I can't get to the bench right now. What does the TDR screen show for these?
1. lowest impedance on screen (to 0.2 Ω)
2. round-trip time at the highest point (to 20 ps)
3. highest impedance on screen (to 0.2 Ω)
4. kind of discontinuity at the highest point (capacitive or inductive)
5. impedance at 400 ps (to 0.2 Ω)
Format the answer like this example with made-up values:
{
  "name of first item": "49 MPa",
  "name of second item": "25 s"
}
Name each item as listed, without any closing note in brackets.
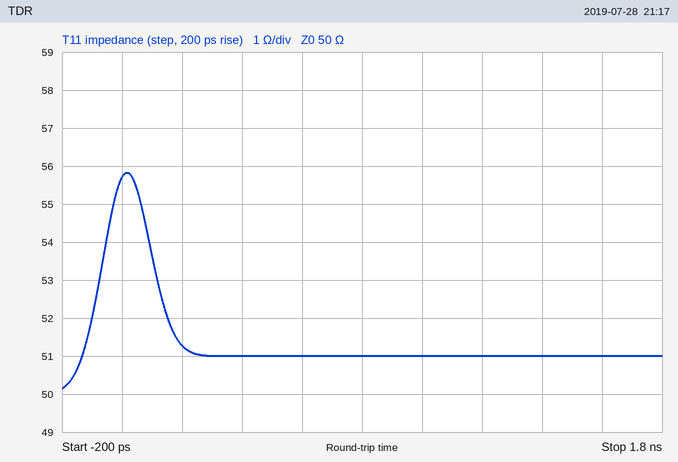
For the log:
{
  "lowest impedance on screen": "50.2 Ω",
  "round-trip time at the highest point": "20 ps",
  "highest impedance on screen": "55.8 Ω",
  "kind of discontinuity at the highest point": "inductive",
  "impedance at 400 ps": "51.0 Ω"
}
